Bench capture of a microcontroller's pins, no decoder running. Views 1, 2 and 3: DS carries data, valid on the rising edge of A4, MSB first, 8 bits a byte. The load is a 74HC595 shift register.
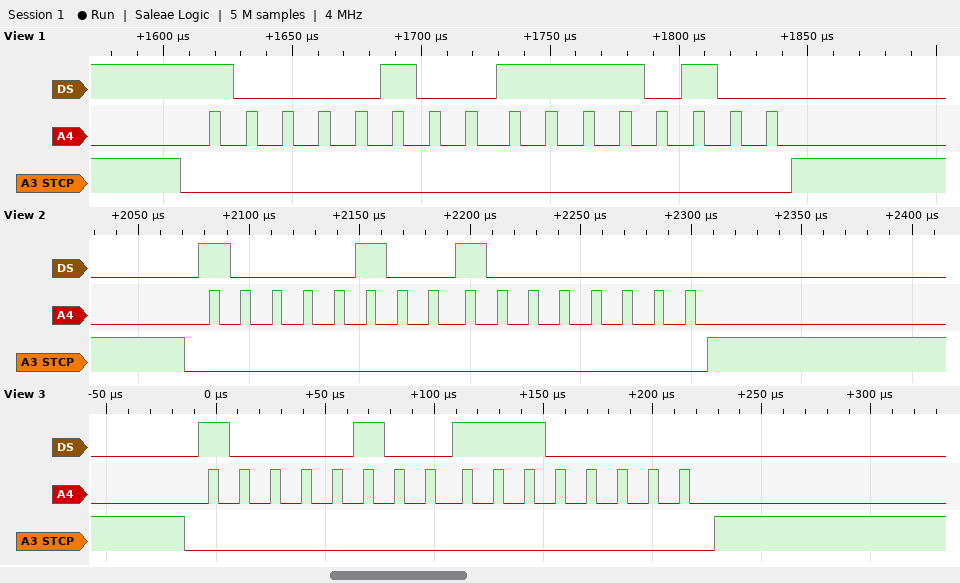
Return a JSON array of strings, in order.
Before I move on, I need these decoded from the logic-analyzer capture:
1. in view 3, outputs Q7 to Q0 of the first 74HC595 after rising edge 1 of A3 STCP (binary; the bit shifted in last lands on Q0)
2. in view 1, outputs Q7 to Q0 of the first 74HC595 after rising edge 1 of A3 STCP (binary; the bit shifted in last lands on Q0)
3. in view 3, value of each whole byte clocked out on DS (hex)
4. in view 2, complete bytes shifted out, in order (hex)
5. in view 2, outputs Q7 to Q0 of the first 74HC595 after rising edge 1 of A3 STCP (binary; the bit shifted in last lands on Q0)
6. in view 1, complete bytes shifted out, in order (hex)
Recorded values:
["11100000", "11110100", "84 E0", "0x84 0x80", "10000000", "84 F4"]
